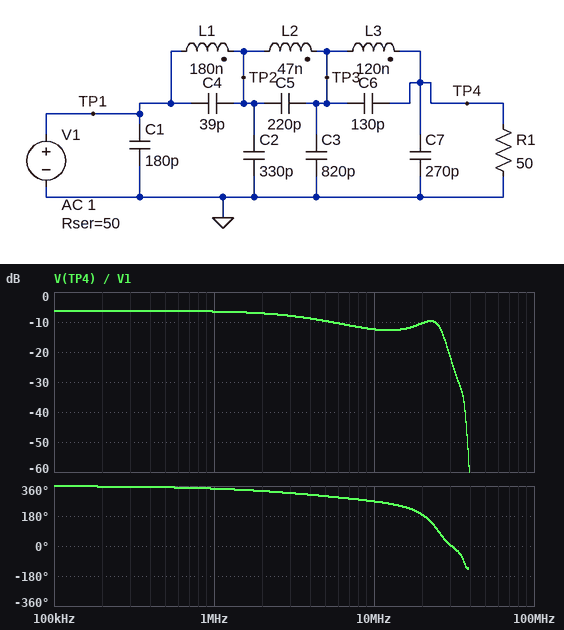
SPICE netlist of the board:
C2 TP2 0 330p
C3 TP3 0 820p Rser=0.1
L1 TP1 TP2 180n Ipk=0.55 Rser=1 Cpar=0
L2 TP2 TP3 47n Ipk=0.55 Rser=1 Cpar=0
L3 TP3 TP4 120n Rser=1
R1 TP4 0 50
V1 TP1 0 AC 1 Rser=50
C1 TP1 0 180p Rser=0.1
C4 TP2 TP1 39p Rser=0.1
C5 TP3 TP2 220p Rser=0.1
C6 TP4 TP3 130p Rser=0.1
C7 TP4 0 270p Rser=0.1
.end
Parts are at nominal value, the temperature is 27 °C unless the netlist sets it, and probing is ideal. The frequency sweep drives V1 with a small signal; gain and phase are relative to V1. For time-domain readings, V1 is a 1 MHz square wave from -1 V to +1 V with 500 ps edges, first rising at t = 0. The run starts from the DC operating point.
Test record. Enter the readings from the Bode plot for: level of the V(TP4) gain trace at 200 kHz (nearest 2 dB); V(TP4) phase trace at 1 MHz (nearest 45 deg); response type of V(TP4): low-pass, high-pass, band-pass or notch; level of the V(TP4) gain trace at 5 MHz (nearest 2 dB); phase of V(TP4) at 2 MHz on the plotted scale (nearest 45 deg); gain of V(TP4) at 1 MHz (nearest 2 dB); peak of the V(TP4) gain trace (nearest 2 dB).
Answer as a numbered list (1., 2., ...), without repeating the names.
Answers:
1. -6 dB
2. 360 deg
3. low-pass
4. -10 dB
5. 315 deg
6. -6 dB
7. -6 dB
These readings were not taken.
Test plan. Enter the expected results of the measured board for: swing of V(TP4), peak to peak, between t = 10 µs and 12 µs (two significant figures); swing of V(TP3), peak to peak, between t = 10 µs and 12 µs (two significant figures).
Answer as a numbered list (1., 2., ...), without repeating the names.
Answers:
1. 970 mV
2. 990 mV
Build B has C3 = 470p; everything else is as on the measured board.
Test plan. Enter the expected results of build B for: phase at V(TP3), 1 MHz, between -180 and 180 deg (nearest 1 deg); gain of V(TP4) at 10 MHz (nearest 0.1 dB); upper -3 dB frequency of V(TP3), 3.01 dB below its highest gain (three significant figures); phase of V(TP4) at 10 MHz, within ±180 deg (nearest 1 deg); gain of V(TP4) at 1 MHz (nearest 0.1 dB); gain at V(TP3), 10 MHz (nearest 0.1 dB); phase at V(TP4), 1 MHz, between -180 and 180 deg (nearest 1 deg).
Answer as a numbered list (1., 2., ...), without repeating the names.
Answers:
1. -12 deg
2. -10.8 dB
3. 5.68 MHz
4. -85 deg
5. -6.4 dB
6. -11.7 dB
7. -13 deg
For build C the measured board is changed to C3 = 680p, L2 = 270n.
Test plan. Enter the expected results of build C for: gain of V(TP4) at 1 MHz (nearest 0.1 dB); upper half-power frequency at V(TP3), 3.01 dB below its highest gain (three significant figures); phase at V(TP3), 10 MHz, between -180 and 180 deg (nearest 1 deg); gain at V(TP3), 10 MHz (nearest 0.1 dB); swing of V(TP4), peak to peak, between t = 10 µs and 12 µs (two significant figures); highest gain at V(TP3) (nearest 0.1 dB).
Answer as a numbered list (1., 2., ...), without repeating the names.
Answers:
1. -6.4 dB
2. 5.73 MHz
3. -103 deg
4. -9.8 dB
5. 1.0 V
6. -6.1 dB
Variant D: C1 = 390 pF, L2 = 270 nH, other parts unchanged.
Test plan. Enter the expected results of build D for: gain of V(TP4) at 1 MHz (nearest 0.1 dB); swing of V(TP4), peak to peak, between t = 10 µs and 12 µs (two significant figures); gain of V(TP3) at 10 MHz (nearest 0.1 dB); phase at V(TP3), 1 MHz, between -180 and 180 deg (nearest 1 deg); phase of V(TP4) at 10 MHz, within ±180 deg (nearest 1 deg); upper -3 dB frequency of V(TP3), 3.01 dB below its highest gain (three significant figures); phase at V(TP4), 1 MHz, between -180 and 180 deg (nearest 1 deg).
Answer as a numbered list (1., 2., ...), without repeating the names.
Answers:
1. -6.5 dB
2. 1.0 V
3. -9.2 dB
4. -17 deg
5. -134 deg
6. 4.49 MHz
7. -18 deg
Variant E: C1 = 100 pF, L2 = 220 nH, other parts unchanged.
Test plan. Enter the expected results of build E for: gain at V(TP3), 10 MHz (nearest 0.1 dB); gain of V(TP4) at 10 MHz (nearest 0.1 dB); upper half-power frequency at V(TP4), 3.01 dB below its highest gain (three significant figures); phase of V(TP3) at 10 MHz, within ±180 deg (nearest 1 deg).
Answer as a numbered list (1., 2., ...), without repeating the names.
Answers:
1. -11.4 dB
2. -10.6 dB
3. 5.33 MHz
4. -95 deg
